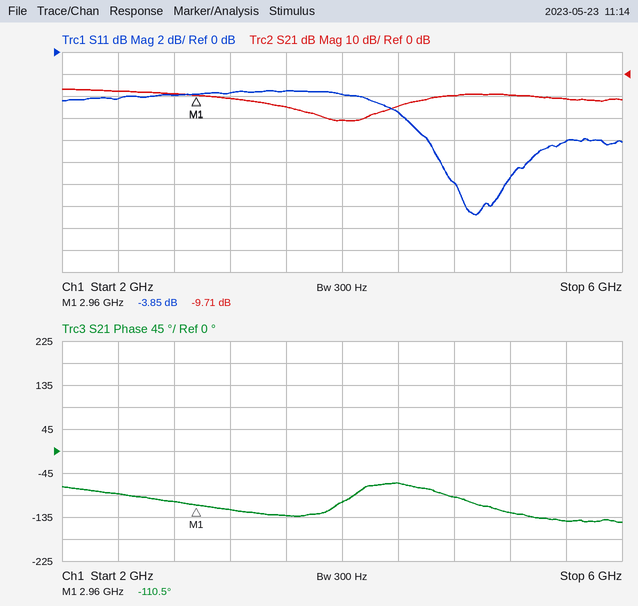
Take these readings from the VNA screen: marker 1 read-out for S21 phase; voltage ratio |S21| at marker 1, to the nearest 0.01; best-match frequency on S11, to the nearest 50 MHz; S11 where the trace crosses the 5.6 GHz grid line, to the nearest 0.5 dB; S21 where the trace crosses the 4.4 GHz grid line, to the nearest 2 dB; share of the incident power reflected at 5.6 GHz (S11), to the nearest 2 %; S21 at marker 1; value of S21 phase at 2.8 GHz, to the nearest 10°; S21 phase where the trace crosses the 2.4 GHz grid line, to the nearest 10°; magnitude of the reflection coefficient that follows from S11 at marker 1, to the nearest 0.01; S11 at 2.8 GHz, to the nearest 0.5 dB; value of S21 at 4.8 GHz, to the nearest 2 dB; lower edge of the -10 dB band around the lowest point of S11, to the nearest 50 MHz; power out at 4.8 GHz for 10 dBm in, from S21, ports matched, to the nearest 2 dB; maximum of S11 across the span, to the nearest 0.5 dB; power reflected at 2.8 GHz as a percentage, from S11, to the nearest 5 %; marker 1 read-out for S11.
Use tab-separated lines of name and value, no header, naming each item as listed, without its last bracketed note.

marker 1 read-out for S21 phase	-110.5°
voltage ratio |S21| at marker 1, to the nearest 0.01	0.33
best-match frequency on S11, to the nearest 50 MHz	4.95 GHz
S11 where the trace crosses the 5.6 GHz grid line, to the nearest 0.5 dB	-8.0 dB
S21 where the trace crosses the 4.4 GHz grid line, to the nearest 2 dB	-14 dB
share of the incident power reflected at 5.6 GHz (S11), to the nearest 2 %	16 %
S21 at marker 1	-9.71 dB
value of S21 phase at 2.8 GHz, to the nearest 10°	-100°
S21 phase where the trace crosses the 2.4 GHz grid line, to the nearest 10°	-90°
magnitude of the reflection coefficient that follows from S11 at marker 1, to the nearest 0.01	0.64
S11 at 2.8 GHz, to the nearest 0.5 dB	-4.0 dB
value of S21 at 4.8 GHz, to the nearest 2 dB	-10 dB
lower edge of the -10 dB band around the lowest point of S11, to the nearest 50 MHz	4.70 GHz
power out at 4.8 GHz for 10 dBm in, from S21, ports matched, to the nearest 2 dB	0 dBm
maximum of S11 across the span, to the nearest 0.5 dB	-3.5 dB
power reflected at 2.8 GHz as a percentage, from S11, to the nearest 5 %	40 %
marker 1 read-out for S11	-3.85 dB
